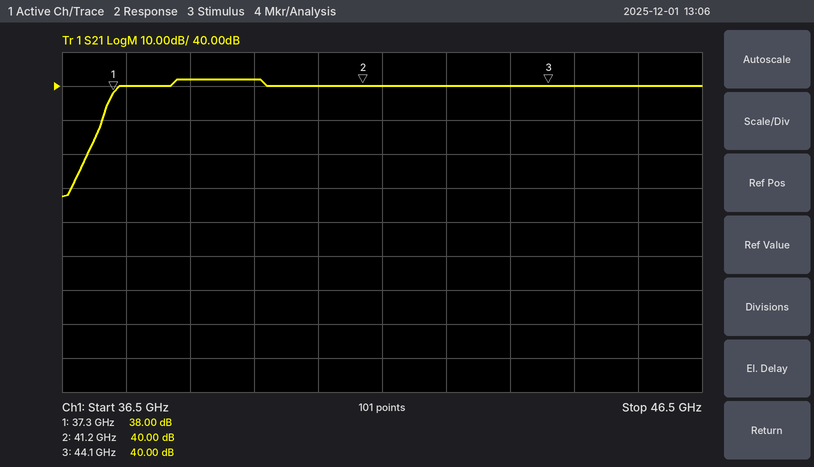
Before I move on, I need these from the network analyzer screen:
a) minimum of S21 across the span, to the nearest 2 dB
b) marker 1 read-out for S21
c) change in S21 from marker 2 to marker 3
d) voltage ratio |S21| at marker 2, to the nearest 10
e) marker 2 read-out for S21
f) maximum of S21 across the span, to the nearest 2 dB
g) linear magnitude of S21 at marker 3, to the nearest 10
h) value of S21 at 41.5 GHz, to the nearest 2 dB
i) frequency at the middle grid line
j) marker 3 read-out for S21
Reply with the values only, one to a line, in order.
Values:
8 dB
38.00 dB
0.00 dB
100
40.00 dB
42 dB
100
40 dB
41.5 GHz
40.00 dB
